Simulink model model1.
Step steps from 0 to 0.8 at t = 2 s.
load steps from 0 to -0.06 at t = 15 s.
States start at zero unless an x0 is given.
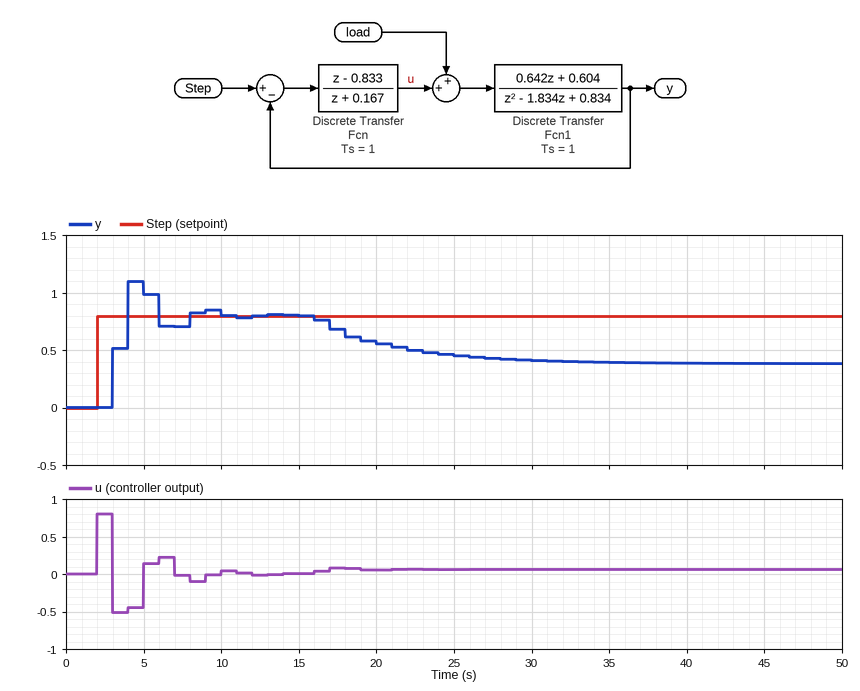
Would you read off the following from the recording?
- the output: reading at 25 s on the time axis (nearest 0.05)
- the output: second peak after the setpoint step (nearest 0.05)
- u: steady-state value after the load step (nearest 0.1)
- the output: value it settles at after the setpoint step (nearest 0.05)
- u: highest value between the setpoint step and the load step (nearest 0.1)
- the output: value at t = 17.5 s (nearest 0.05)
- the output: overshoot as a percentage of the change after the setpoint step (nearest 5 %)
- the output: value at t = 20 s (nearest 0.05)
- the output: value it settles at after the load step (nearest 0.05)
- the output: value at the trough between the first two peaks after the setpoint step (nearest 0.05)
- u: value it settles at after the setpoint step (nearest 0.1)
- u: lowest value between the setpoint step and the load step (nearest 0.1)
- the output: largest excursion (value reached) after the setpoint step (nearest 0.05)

0.45
0.85
0.1
0.80
0.8
0.70
35 %
0.55
0.40
0.70
0.0
-0.5
1.10
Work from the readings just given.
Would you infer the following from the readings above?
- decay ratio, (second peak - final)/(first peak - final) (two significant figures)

0.17
